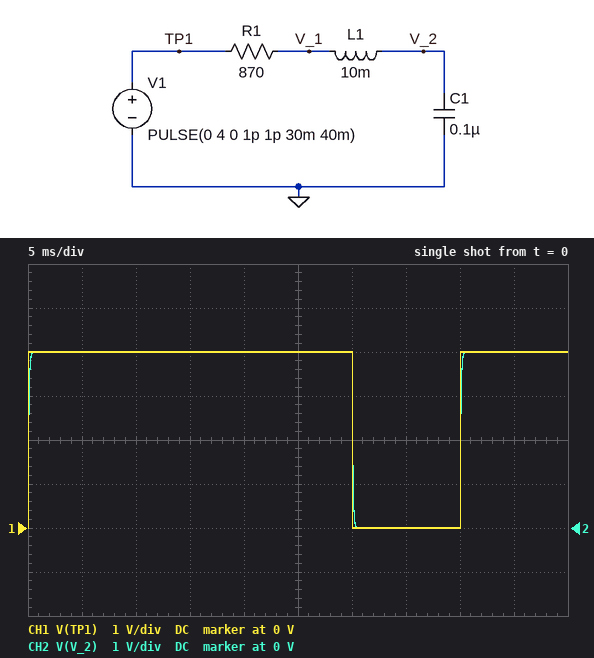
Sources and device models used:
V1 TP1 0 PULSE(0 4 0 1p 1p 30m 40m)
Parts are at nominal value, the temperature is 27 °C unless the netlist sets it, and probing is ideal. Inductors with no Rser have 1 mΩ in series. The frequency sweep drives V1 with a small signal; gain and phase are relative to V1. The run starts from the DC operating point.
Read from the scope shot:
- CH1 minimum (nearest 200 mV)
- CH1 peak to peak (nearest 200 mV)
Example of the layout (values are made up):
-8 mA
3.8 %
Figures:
0 V
4.0 V
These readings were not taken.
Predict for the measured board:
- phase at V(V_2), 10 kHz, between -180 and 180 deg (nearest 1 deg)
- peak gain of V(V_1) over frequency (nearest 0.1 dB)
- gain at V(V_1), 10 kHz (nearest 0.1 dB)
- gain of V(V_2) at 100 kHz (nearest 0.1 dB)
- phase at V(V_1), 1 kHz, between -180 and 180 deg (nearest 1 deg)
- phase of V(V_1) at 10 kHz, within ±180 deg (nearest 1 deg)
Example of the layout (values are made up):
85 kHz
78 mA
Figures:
-118 deg
0 dB
-6.5 dB
-52.0 dB
-30 deg
62 deg
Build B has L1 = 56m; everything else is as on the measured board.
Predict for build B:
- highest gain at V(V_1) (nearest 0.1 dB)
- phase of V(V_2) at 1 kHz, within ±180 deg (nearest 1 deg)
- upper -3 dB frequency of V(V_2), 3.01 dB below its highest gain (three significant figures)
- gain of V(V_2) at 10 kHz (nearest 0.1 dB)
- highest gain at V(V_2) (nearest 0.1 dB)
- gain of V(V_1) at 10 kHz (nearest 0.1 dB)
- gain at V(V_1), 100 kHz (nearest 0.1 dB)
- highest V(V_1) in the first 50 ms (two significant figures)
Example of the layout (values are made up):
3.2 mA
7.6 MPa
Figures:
0 dB
-35 deg
2.40 kHz
-26.8 dB
0.5 dB
-0.3 dB
0 dB
4.3 V
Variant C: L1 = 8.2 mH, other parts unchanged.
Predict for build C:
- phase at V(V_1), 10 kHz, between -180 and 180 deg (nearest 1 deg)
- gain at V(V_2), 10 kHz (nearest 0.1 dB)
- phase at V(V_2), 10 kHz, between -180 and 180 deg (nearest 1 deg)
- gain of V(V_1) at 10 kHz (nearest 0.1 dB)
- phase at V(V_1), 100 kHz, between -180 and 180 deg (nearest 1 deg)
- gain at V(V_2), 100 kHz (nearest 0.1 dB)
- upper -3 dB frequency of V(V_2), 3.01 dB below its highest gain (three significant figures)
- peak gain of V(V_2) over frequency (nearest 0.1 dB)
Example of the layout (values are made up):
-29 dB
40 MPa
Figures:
68 deg
-15.4 dB
-112 deg
-8.4 dB
10 deg
-50.3 dB
2.05 kHz
0 dB
